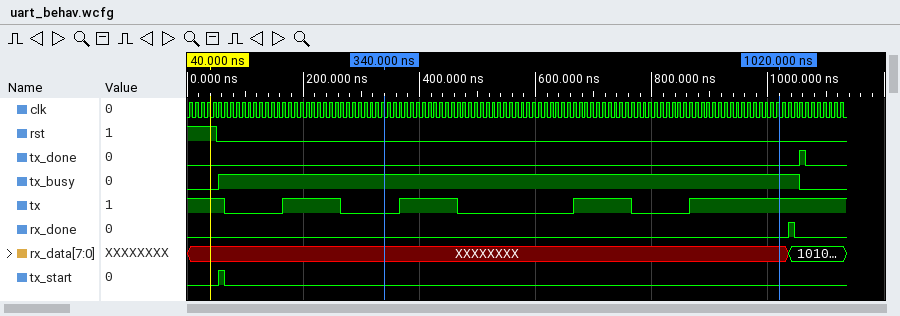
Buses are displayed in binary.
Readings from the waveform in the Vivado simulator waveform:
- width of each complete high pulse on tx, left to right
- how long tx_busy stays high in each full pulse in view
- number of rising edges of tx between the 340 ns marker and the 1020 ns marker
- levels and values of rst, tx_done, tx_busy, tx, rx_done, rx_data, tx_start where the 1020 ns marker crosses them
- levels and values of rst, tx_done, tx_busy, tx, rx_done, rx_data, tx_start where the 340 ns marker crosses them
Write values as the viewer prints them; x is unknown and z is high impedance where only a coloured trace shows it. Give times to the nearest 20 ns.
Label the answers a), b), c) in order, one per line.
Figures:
a) 100 ns, 100 ns, 100 ns
b) 1000 ns
c) 3
d) rst=0, tx_done=0, tx_busy=1, tx=1, rx_done=0, rx_data=XXXXXXXX, tx_start=0
e) rst=0, tx_done=0, tx_busy=1, tx=0, rx_done=0, rx_data=XXXXXXXX, tx_start=0
